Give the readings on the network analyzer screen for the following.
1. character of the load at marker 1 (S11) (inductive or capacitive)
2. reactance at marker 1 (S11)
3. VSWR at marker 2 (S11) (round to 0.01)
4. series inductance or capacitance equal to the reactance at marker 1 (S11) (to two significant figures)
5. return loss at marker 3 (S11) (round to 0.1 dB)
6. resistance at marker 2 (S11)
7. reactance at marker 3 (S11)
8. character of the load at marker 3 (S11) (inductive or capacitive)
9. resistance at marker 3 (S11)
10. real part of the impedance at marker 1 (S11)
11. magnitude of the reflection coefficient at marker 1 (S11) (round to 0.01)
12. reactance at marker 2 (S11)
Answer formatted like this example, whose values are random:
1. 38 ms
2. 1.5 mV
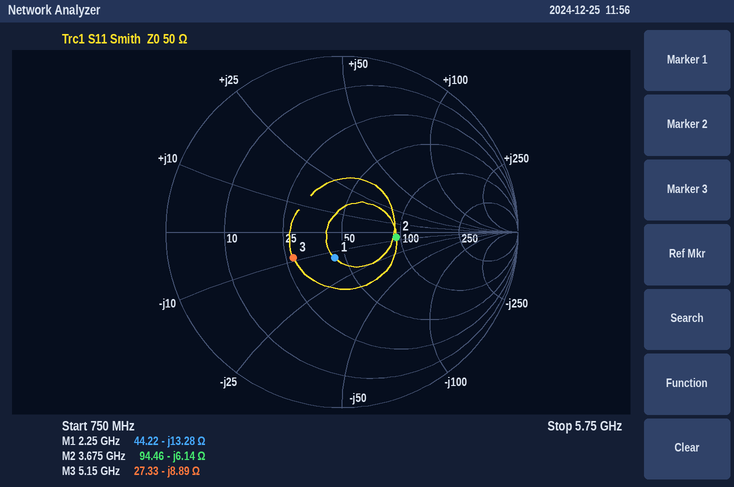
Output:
1. capacitive
2. -13.28 Ω
3. 1.90
4. 5.3 pF
5. 10.1 dB
6. 94.46 Ω
7. -8.89 Ω
8. capacitive
9. 27.33 Ω
10. 44.22 Ω
11. 0.15
12. -6.14 Ω
